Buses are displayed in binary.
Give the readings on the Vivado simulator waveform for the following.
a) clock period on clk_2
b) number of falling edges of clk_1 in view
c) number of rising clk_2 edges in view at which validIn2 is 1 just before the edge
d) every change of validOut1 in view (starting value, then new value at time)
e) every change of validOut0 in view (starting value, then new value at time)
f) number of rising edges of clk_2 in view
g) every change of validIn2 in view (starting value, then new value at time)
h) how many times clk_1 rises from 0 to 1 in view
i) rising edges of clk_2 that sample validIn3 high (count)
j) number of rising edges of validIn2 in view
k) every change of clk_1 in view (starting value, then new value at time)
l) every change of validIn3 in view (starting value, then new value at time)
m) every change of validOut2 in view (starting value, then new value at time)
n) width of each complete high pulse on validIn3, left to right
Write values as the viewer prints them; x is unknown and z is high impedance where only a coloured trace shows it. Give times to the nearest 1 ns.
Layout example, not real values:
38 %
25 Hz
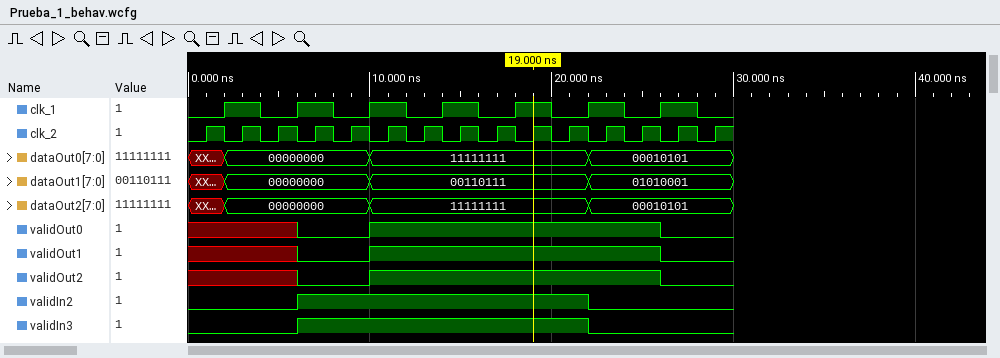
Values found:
2 ns
7
8
x, 0 at 6 ns, 1 at 10 ns, 0 at 26 ns
x, 0 at 6 ns, 1 at 10 ns, 0 at 26 ns
15
0, 1 at 6 ns, 0 at 22 ns
7
8
1
0, 1 at 2 ns, 0 at 4 ns, 1 at 6 ns, 0 at 8 ns, 1 at 10 ns, 0 at 12 ns, 1 at 14 ns, 0 at 16 ns, 1 at 18 ns, 0 at 20 ns, 1 at 22 ns, 0 at 24 ns, 1 at 26 ns, 0 at 28 ns
0, 1 at 6 ns, 0 at 22 ns
x, 0 at 6 ns, 1 at 10 ns, 0 at 26 ns
16 ns
